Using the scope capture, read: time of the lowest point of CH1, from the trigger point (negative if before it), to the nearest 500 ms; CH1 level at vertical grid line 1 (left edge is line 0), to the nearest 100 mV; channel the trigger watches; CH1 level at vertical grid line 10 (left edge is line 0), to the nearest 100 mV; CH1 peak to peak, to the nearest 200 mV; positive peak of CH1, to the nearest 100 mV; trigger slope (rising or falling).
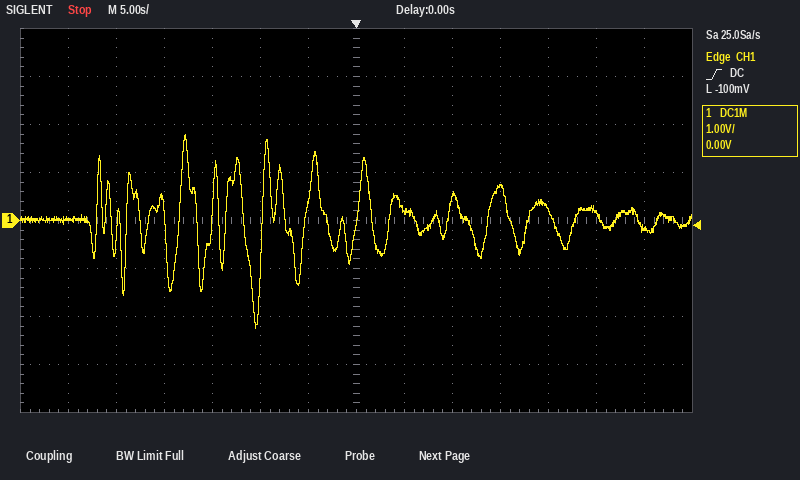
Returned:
-10.5 s
0.0 V
CH1
700 mV
4.0 V
1.8 V
rising
